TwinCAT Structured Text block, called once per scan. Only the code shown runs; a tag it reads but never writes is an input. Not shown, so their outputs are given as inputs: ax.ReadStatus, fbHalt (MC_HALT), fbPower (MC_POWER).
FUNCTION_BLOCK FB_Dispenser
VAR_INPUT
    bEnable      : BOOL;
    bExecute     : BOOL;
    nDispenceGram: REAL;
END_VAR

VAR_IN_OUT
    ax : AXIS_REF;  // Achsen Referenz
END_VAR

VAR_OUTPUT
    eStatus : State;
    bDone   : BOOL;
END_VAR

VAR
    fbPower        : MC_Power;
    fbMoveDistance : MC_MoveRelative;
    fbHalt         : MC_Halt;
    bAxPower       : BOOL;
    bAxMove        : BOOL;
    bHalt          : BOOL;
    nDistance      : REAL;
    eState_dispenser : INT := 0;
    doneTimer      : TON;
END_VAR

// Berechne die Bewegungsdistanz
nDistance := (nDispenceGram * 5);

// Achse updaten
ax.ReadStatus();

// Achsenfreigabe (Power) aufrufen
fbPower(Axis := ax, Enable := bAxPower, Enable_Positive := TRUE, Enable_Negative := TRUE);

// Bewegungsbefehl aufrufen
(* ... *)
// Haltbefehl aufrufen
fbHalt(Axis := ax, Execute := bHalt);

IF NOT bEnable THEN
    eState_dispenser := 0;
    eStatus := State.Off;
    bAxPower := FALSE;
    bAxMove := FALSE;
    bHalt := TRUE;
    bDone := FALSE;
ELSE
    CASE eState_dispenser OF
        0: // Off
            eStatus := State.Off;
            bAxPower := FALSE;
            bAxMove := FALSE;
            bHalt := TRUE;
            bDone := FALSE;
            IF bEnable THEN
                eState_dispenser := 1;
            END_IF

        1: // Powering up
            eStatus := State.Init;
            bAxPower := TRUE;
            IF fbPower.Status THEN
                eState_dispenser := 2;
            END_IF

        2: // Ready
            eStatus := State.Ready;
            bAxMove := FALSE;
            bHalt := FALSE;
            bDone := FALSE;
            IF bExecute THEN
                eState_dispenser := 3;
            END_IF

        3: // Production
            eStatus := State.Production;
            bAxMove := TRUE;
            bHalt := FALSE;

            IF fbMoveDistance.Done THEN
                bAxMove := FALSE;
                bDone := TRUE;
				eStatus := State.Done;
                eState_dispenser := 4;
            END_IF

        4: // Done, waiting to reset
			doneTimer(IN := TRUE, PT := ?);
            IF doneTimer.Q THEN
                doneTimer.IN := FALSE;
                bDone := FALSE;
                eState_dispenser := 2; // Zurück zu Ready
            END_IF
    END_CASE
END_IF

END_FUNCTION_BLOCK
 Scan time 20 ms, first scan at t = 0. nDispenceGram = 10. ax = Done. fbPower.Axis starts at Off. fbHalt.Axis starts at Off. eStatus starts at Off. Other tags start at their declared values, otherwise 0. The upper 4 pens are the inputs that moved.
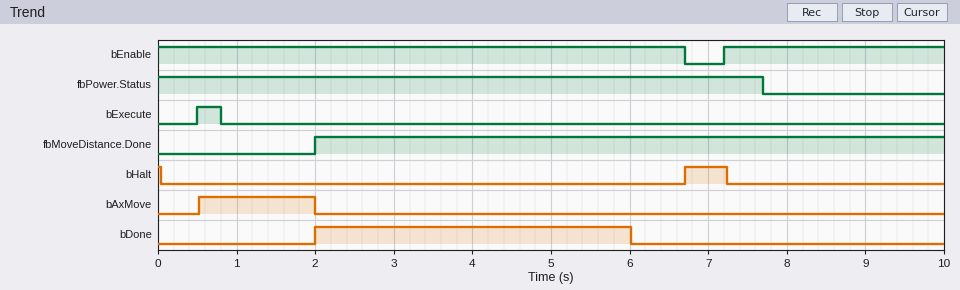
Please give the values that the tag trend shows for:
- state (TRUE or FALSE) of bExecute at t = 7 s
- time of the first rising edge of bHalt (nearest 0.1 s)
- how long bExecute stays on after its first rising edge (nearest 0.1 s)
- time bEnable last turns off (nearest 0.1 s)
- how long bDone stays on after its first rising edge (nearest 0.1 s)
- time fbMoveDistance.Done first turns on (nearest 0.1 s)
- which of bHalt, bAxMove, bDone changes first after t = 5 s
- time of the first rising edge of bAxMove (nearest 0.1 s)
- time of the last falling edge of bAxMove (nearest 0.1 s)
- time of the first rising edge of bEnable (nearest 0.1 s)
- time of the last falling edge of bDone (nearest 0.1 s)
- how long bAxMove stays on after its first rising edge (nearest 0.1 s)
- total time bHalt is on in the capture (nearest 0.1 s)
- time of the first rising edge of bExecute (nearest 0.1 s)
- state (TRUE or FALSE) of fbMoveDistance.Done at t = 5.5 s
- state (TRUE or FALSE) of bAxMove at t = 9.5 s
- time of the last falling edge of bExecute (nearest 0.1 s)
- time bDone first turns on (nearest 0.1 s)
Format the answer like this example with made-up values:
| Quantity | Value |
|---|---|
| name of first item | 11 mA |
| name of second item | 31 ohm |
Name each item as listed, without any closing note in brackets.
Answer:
| Quantity | Value |
|---|---|
| state (TRUE or FALSE) of bExecute at t = 7 s | FALSE |
| time of the first rising edge of bHalt | 6.7 s |
| how long bExecute stays on after its first rising edge | 0.3 s |
| time bEnable last turns off | 6.7 s |
| how long bDone stays on after its first rising edge | 4.0 s |
| time fbMoveDistance.Done first turns on | 2.0 s |
| which of bHalt, bAxMove, bDone changes first after t = 5 s | bDone |
| time of the first rising edge of bAxMove | 0.5 s |
| time of the last falling edge of bAxMove | 2.0 s |
| time of the first rising edge of bEnable | 7.2 s |
| time of the last falling edge of bDone | 6.0 s |
| how long bAxMove stays on after its first rising edge | 1.5 s |
| total time bHalt is on in the capture | 0.6 s |
| time of the first rising edge of bExecute | 0.5 s |
| state (TRUE or FALSE) of fbMoveDistance.Done at t = 5.5 s | TRUE |
| state (TRUE or FALSE) of bAxMove at t = 9.5 s | FALSE |
| time of the last falling edge of bExecute | 0.8 s |
| time bDone first turns on | 2.0 s |
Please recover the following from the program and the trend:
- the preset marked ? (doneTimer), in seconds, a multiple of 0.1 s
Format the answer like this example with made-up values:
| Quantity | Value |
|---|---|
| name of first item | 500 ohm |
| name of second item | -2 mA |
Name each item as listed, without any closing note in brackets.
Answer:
| Quantity | Value |
|---|---|
| the preset marked ? (doneTimer), in seconds, a multiple of 0.1 s | 4.0 s |
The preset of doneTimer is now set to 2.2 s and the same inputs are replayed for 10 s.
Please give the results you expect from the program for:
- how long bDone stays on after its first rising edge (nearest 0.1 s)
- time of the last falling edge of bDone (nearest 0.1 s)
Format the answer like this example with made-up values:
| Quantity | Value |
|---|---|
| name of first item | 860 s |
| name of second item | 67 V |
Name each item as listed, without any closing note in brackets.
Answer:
| Quantity | Value |
|---|---|
| how long bDone stays on after its first rising edge | 2.2 s |
| time of the last falling edge of bDone | 4.2 s |
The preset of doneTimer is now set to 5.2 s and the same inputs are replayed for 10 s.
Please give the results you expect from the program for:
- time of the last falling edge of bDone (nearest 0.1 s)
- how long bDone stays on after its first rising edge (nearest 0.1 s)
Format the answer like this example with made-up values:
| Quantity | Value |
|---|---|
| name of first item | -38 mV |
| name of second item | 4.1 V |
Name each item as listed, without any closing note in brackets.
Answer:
| Quantity | Value |
|---|---|
| time of the last falling edge of bDone | 6.7 s |
| how long bDone stays on after its first rising edge | 4.7 s |
